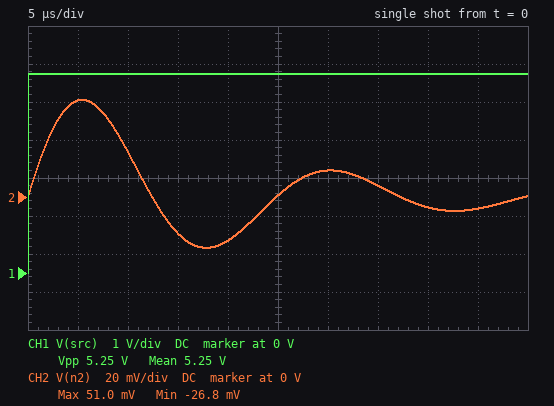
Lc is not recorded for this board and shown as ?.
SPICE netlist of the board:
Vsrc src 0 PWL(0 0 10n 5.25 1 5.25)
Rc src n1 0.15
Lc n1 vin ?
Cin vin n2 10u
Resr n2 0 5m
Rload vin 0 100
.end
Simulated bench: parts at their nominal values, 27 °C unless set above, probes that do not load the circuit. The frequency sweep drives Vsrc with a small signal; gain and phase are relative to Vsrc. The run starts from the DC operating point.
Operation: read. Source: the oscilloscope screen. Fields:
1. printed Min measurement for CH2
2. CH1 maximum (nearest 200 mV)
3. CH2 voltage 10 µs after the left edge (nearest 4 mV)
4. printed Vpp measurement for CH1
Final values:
-26.8 mV
5.2 V
24 mV
5.25 V
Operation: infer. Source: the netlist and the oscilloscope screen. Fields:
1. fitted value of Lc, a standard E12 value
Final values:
1.5 µH
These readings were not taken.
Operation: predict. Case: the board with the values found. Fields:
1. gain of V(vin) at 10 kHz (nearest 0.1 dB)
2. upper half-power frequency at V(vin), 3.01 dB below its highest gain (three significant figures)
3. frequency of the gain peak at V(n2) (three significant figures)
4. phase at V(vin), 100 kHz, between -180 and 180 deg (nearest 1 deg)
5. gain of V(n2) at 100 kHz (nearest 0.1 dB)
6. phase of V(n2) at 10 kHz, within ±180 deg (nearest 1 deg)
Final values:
0.5 dB
47.1 kHz
41.1 kHz
-167 deg
-44.1 dB
84 deg
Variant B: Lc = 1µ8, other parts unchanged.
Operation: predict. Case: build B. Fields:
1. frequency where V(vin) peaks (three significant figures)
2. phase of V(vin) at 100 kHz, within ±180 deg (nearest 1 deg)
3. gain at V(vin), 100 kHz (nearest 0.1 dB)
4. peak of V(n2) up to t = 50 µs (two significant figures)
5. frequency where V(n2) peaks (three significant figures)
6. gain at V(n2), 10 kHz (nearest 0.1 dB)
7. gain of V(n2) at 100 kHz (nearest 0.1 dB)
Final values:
36.2 kHz
-169 deg
-15.8 dB
48 mV
37.5 kHz
-49.5 dB
-45.9 dB
